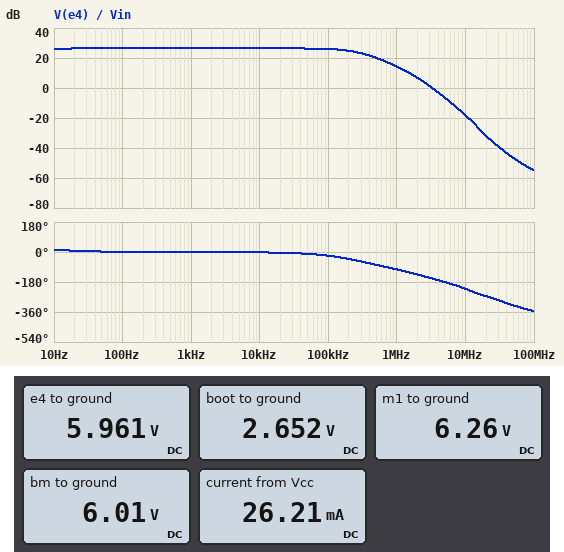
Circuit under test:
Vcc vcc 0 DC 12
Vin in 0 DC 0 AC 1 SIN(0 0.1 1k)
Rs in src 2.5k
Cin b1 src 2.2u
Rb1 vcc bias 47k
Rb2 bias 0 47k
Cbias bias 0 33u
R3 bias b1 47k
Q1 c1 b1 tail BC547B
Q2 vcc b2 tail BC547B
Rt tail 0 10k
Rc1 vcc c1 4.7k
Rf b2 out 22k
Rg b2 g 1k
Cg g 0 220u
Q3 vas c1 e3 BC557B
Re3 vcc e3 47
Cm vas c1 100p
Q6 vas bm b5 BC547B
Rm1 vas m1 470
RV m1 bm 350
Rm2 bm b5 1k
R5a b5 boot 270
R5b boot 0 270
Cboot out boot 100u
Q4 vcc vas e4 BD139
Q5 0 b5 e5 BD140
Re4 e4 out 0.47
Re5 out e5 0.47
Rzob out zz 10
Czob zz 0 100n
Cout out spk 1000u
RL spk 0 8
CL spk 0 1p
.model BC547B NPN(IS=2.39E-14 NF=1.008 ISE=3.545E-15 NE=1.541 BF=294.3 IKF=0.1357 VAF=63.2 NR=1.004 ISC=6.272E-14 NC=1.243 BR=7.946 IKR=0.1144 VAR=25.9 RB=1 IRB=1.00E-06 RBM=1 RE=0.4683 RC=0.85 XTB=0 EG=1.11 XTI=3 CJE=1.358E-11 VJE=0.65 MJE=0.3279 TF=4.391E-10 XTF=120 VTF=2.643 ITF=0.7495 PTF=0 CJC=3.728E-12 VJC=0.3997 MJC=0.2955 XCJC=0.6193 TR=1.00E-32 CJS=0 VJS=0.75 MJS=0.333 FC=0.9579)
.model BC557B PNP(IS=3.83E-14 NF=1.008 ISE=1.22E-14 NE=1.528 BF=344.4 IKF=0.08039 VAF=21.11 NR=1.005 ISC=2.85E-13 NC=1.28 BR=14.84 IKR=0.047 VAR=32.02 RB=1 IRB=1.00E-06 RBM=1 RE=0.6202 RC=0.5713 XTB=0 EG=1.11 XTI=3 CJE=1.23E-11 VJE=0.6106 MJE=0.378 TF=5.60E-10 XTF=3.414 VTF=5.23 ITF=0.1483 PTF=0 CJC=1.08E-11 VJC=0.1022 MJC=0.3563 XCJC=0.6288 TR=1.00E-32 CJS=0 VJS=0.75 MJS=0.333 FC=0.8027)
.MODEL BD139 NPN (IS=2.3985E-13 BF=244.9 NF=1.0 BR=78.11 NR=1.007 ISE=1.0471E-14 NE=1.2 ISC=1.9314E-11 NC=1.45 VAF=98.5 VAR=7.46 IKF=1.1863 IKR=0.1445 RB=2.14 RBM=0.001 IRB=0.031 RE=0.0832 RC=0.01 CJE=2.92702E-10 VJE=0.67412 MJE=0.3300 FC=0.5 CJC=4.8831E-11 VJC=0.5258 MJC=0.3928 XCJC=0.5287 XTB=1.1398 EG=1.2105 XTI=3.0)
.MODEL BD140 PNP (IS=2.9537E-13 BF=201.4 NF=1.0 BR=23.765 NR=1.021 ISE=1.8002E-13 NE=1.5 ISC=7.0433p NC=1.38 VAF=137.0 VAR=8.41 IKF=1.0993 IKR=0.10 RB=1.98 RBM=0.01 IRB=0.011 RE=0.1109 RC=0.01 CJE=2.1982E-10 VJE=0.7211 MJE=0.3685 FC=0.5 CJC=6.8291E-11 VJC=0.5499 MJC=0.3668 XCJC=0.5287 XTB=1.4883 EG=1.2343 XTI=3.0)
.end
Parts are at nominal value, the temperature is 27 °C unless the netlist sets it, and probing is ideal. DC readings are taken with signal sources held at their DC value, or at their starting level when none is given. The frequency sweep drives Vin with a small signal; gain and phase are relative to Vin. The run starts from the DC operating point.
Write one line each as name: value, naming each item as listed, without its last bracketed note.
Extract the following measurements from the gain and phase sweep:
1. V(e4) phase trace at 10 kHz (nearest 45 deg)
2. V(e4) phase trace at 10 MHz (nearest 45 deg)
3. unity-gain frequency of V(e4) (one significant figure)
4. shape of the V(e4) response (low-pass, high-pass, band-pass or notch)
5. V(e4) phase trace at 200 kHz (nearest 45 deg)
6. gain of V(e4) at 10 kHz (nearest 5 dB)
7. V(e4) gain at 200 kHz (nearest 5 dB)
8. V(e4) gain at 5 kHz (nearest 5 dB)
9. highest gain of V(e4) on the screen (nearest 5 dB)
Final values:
V(e4) phase trace at 10 kHz: 0 deg
V(e4) phase trace at 10 MHz: -225 deg
unity-gain frequency of V(e4): 3 MHz
shape of the V(e4) response: low-pass
V(e4) phase trace at 200 kHz: -45 deg
gain of V(e4) at 10 kHz: 25 dB
V(e4) gain at 200 kHz: 25 dB
V(e4) gain at 5 kHz: 25 dB
highest gain of V(e4) on the screen: 25 dB
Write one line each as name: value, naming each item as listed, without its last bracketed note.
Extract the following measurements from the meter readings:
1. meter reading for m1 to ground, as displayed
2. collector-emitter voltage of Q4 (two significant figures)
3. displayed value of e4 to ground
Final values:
meter reading for m1 to ground, as displayed: 6.26 V
collector-emitter voltage of Q4: 6.0 V
displayed value of e4 to ground: 5.961 V
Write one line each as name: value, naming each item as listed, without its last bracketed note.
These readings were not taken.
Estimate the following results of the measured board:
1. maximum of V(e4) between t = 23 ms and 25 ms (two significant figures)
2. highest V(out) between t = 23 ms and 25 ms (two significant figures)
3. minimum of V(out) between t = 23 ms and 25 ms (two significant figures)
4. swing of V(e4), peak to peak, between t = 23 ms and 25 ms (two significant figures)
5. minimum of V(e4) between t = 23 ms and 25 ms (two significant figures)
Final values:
maximum of V(e4) between t = 23 ms and 25 ms: 8.1 V
highest V(out) between t = 23 ms and 25 ms: 8.0 V
minimum of V(out) between t = 23 ms and 25 ms: 3.9 V
swing of V(e4), peak to peak, between t = 23 ms and 25 ms: 4.2 V
minimum of V(e4) between t = 23 ms and 25 ms: 3.9 V
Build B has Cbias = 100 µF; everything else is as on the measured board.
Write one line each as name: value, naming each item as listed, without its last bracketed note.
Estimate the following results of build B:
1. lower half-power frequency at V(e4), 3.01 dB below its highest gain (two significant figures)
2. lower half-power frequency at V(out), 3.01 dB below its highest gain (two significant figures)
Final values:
lower half-power frequency at V(e4), 3.01 dB below its highest gain: 2.1 Hz
lower half-power frequency at V(out), 3.01 dB below its highest gain: 2.0 Hz
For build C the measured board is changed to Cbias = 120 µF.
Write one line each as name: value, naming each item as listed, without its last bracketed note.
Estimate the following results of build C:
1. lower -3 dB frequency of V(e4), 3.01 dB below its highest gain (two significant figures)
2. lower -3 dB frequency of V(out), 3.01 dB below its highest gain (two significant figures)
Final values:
lower -3 dB frequency of V(e4), 3.01 dB below its highest gain: 2.1 Hz
lower -3 dB frequency of V(out), 3.01 dB below its highest gain: 2.0 Hz
